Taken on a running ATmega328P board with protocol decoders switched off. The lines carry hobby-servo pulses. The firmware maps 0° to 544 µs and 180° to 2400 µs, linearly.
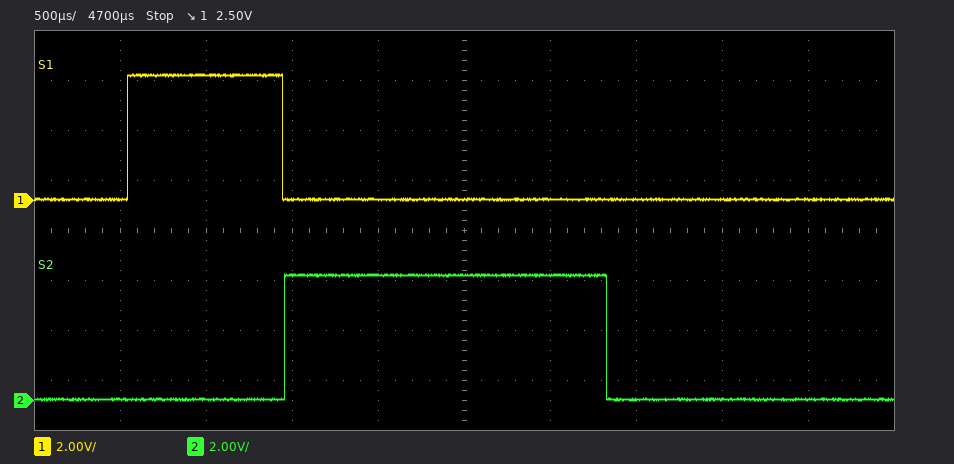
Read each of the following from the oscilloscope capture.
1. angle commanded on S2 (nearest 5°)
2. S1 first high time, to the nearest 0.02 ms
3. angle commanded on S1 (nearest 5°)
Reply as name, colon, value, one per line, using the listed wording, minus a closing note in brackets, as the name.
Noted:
angle commanded on S2: 130°
S1 first high time, to the nearest 0.02 ms: 0.90 ms
angle commanded on S1: 35°
